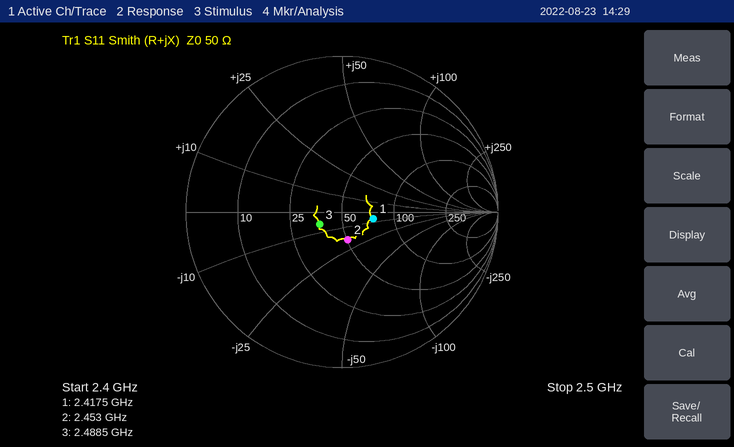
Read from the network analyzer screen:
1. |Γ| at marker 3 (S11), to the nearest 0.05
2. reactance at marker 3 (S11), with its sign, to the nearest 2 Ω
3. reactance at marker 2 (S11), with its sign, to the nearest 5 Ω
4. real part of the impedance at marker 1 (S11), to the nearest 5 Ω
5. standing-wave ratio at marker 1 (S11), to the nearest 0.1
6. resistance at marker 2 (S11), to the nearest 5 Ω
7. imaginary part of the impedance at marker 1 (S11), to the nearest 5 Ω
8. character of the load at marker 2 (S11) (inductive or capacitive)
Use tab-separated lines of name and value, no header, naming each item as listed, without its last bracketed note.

|Γ| at marker 3 (S11), to the nearest 0.05	0.15
reactance at marker 3 (S11), with its sign, to the nearest 2 Ω	-6 Ω
reactance at marker 2 (S11), with its sign, to the nearest 5 Ω	-20 Ω
real part of the impedance at marker 1 (S11), to the nearest 5 Ω	75 Ω
standing-wave ratio at marker 1 (S11), to the nearest 0.1	1.5
resistance at marker 2 (S11), to the nearest 5 Ω	50 Ω
imaginary part of the impedance at marker 1 (S11), to the nearest 5 Ω	-5 Ω
character of the load at marker 2 (S11)	capacitive
